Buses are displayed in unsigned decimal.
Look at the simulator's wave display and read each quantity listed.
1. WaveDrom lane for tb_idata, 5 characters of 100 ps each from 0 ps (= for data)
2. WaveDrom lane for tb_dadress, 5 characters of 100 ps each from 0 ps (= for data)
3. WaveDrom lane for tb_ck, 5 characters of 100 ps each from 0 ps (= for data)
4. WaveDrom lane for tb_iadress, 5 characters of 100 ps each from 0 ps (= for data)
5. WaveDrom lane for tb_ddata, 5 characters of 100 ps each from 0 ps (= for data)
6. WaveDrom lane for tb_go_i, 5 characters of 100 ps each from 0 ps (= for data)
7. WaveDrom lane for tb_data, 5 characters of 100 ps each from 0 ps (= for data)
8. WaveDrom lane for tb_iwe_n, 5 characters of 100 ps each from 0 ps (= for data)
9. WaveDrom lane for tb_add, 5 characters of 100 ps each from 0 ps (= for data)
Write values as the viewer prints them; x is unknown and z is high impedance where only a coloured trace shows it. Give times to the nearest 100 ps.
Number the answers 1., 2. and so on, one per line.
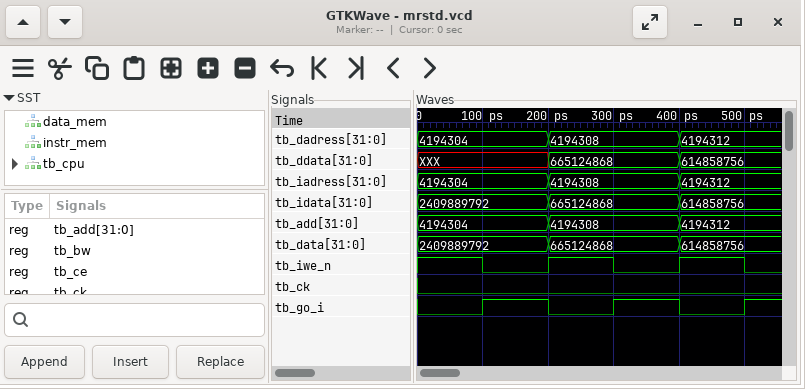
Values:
1. {name: 'tb_idata', wave: '=.=.=', data: '2409889792 665124868 614858756'}
2. {name: 'tb_dadress', wave: '=.=.=', data: '4194304 4194308 4194312'}
3. {name: 'tb_ck', wave: '0....'}
4. {name: 'tb_iadress', wave: '=.=.=', data: '4194304 4194308 4194312'}
5. {name: 'tb_ddata', wave: 'x.=.=', data: '665124868 614858756'}
6. {name: 'tb_go_i', wave: '01010'}
7. {name: 'tb_data', wave: '=.=.=', data: '2409889792 665124868 614858756'}
8. {name: 'tb_iwe_n', wave: '10101'}
9. {name: 'tb_add', wave: '=.=.=', data: '4194304 4194308 4194312'}
